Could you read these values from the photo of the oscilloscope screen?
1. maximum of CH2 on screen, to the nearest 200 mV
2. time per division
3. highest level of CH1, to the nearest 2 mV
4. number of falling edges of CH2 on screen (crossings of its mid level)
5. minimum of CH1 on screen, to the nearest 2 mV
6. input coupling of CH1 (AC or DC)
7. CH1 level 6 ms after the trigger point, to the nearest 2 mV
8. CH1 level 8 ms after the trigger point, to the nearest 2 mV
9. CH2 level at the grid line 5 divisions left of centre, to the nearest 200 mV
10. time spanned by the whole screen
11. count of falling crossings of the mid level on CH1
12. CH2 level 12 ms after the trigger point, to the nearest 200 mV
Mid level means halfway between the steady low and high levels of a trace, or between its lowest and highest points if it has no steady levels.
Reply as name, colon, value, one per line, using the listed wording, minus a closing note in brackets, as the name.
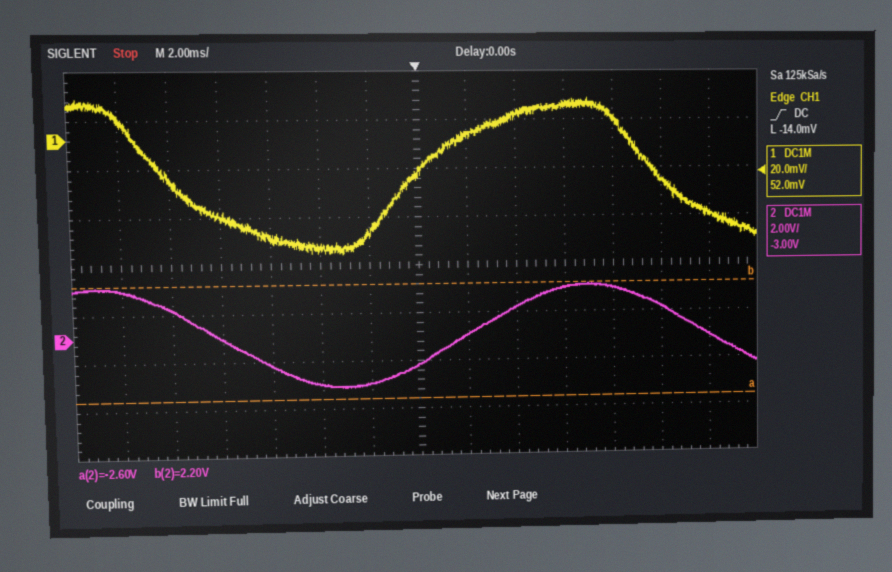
maximum of CH2 on screen, to the nearest 200 mV: 2.2 V
time per division: 2 ms
highest level of CH1, to the nearest 2 mV: 16 mV
number of falling edges of CH2 on screen: 2
minimum of CH1 on screen, to the nearest 2 mV: -46 mV
input coupling of CH1: DC
CH1 level 6 ms after the trigger point, to the nearest 2 mV: 14 mV
CH1 level 8 ms after the trigger point, to the nearest 2 mV: 8 mV
CH2 level at the grid line 5 divisions left of centre, to the nearest 200 mV: 1.2 V
time spanned by the whole screen: 28 ms
count of falling crossings of the mid level on CH1: 2
CH2 level 12 ms after the trigger point, to the nearest 200 mV: 0.0 V
